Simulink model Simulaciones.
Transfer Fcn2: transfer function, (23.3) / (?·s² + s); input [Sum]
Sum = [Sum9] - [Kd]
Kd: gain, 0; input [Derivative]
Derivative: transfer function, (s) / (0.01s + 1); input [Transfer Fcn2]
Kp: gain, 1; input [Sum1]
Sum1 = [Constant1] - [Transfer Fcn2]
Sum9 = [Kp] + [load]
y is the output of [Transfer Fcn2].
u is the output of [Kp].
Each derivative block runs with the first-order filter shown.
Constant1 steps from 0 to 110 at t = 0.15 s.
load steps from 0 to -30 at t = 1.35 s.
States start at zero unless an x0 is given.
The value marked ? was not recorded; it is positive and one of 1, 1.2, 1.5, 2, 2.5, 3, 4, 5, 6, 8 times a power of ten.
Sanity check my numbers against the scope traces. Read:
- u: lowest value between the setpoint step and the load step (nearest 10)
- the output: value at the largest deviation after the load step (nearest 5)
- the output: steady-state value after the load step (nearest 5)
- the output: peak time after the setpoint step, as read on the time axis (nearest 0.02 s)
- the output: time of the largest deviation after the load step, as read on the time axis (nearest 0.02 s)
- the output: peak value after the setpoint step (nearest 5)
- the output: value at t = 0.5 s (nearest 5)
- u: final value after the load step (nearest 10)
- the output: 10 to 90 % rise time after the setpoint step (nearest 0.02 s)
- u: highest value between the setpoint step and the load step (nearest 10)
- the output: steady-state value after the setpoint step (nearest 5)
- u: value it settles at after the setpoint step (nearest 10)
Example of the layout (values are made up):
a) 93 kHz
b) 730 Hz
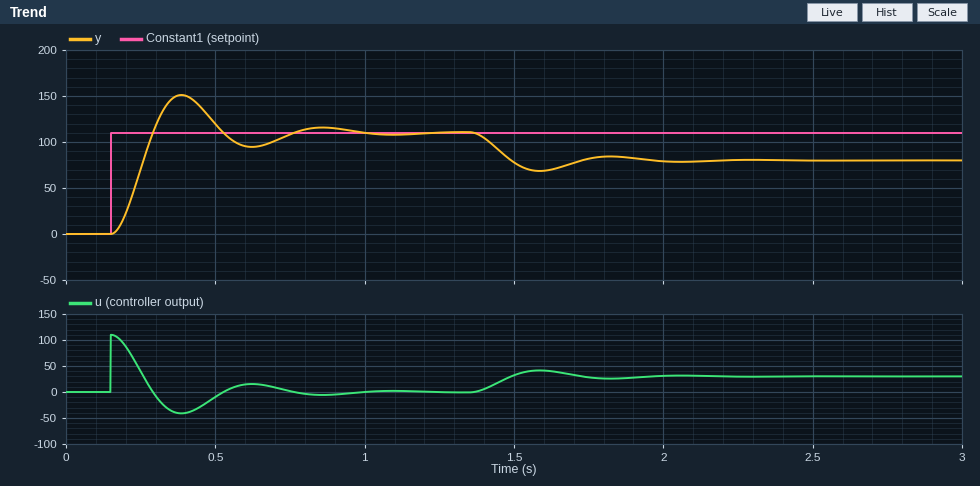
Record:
a) -40
b) 70
c) 80
d) 0.38 s
e) 1.58 s
f) 150
g) 120
h) 30
i) 0.10 s
j) 110
k) 110
l) 0
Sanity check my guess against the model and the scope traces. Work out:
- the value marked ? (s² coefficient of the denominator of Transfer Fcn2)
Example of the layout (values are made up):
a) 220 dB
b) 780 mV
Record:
a) 0.12
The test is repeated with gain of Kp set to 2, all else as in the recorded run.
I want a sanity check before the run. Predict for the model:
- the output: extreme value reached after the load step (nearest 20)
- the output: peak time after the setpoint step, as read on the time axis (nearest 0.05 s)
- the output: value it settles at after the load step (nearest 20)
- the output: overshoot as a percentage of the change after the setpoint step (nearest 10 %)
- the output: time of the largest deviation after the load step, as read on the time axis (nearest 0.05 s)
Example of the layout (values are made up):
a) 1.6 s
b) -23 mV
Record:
a) 80
b) 0.30 s
c) 100
d) 50 %
e) 1.50 s
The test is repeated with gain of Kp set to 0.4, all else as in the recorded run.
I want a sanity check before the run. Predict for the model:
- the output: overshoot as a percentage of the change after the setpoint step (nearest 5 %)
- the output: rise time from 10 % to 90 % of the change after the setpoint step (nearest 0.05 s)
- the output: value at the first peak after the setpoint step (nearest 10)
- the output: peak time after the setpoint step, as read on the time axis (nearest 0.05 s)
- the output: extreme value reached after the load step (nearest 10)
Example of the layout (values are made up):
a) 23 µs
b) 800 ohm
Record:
a) 20 %
b) 0.20 s
c) 130
d) 0.55 s
e) 20
